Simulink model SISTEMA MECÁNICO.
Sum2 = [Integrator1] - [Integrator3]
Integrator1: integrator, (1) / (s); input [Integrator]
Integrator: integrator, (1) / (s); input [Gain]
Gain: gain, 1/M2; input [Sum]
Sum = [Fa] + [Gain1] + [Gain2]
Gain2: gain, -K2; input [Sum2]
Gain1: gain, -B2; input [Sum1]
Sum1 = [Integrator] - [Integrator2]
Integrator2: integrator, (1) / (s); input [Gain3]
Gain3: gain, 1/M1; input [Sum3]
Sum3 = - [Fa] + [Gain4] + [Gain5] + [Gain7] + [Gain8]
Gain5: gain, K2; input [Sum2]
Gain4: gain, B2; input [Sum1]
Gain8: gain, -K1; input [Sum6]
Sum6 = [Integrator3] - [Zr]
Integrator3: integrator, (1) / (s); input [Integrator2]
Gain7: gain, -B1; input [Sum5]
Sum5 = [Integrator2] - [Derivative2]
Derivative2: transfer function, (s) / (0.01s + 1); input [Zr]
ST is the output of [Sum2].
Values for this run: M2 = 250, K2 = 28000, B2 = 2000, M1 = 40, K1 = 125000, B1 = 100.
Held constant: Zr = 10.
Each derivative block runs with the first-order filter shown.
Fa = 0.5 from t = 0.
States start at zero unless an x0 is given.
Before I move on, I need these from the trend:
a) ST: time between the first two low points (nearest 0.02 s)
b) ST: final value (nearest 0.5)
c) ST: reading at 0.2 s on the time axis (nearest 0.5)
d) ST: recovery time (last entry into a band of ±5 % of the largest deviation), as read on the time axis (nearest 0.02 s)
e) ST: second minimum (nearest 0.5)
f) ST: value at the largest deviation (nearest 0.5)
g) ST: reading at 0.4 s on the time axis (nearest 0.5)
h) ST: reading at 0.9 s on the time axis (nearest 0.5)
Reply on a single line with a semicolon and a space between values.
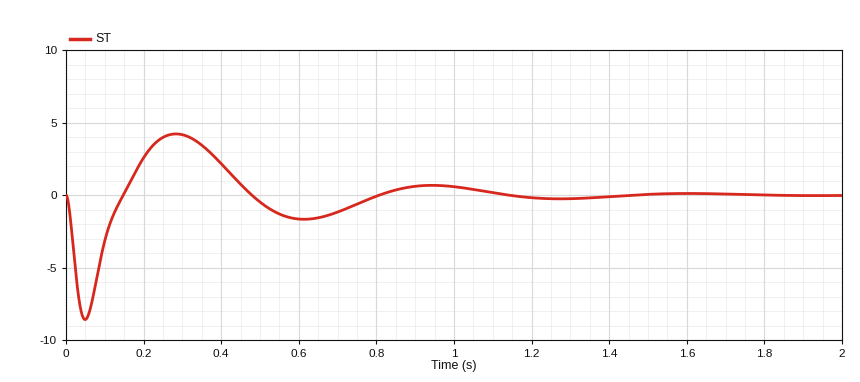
0.56 s; 0.0; 2.5; 1.04 s; -1.5; -8.5; 2.0; 0.5
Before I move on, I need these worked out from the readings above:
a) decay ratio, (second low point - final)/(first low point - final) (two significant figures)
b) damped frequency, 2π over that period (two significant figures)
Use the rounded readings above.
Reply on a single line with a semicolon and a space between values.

0.18; 11 rad/s
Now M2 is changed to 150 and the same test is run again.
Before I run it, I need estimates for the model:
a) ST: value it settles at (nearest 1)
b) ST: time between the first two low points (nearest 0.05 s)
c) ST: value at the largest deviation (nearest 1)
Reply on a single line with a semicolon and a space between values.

0; 0.40 s; -8
